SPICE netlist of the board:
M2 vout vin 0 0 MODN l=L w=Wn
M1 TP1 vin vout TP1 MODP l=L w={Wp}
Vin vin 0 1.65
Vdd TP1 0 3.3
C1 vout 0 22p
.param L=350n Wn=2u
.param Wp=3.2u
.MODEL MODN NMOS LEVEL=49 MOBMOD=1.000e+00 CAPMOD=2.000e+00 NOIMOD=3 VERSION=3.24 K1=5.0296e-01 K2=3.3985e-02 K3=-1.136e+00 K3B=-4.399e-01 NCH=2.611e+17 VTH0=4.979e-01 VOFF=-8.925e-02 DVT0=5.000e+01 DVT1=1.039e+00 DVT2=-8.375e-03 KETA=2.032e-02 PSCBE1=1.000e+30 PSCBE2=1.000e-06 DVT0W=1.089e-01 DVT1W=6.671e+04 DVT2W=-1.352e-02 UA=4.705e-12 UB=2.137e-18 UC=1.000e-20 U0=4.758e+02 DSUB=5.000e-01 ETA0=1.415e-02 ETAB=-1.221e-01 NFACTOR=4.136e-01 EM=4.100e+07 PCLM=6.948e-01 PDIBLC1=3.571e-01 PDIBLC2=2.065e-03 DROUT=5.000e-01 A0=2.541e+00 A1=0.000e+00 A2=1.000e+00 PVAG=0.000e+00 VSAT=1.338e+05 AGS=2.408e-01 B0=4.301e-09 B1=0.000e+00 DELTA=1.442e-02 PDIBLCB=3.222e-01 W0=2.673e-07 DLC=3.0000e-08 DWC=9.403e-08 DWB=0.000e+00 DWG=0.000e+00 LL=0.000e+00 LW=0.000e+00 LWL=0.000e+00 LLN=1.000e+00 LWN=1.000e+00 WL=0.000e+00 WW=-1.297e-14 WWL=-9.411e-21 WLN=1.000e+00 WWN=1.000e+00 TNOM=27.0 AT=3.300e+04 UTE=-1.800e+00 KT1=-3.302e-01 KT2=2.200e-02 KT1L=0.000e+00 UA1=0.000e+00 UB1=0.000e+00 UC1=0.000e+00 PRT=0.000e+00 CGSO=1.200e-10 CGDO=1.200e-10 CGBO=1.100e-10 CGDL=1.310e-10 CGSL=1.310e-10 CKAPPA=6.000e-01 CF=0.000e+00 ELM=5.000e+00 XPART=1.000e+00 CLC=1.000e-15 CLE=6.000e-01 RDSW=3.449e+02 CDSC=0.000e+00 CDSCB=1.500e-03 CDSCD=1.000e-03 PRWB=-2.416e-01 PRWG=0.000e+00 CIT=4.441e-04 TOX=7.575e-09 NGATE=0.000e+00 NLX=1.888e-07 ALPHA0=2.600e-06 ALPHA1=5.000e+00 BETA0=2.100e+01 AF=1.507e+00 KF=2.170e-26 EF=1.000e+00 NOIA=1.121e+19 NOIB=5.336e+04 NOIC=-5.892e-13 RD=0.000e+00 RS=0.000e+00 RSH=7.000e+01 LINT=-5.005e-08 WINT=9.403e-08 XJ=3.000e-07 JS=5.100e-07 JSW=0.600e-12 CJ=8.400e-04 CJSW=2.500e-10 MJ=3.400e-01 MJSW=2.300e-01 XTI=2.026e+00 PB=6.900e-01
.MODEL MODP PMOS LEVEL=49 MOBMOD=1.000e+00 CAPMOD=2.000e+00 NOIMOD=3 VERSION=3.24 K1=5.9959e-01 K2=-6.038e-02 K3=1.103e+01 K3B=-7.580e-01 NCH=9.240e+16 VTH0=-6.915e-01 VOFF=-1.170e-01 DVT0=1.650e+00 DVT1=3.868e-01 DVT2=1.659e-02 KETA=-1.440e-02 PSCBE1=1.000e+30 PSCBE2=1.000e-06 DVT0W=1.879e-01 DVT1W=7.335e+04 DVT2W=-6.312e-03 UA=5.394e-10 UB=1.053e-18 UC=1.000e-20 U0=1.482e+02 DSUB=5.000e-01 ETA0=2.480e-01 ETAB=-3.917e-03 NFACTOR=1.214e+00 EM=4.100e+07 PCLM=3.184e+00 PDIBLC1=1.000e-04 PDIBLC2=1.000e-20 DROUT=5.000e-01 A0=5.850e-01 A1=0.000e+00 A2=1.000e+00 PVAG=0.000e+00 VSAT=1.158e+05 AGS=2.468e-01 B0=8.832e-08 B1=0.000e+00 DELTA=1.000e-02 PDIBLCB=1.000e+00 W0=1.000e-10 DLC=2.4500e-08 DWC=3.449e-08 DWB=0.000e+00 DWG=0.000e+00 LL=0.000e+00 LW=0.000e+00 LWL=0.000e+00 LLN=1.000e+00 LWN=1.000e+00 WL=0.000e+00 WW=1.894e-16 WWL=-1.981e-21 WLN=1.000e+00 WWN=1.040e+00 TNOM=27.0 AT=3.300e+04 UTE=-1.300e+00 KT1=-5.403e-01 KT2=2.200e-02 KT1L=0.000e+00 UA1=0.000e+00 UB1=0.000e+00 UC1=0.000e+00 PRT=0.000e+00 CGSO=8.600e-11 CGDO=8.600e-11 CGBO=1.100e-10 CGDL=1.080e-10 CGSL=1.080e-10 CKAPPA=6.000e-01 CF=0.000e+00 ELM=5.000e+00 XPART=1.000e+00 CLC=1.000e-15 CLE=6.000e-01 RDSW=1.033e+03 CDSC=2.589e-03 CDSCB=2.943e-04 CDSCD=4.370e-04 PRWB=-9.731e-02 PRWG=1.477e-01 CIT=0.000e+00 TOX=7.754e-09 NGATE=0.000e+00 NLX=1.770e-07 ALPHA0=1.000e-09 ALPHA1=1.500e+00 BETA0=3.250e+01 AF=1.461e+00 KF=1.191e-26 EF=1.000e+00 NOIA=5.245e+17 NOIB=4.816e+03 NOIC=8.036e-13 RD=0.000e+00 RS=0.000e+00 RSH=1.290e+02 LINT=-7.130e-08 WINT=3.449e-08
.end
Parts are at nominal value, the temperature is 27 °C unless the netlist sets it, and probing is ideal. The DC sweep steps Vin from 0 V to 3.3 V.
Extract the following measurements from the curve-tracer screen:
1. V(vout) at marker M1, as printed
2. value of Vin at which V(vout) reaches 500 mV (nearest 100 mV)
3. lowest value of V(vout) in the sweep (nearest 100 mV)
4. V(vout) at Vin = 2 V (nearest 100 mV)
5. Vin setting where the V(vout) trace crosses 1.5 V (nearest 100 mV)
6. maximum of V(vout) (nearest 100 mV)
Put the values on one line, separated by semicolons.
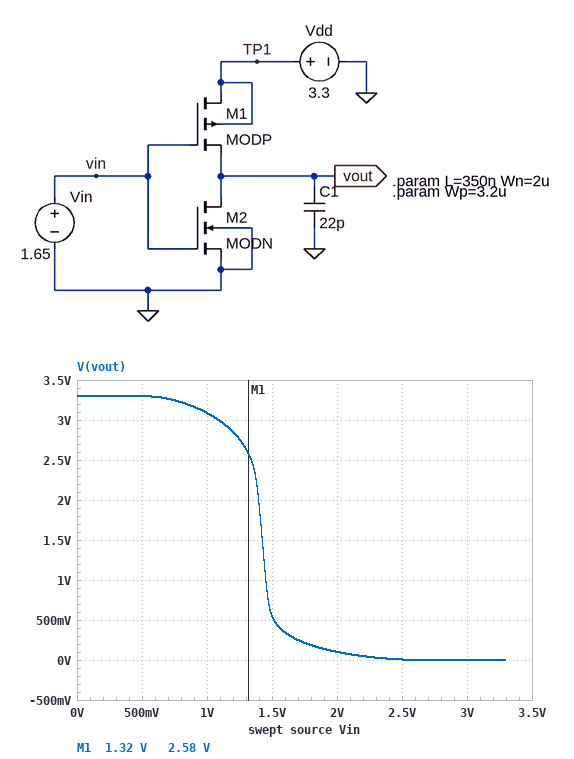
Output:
2.58 V; 1.5 V; 0 V; 100 mV; 1.4 V; 3.3 V
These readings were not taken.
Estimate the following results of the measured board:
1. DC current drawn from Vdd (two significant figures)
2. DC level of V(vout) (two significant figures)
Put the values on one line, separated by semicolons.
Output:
150 µA; 290 mV
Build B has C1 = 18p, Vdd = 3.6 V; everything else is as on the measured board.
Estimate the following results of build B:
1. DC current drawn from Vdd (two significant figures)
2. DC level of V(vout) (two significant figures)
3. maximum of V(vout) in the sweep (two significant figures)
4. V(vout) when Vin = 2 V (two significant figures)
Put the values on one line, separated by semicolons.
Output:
230 µA; 590 mV; 3.6 V; 210 mV
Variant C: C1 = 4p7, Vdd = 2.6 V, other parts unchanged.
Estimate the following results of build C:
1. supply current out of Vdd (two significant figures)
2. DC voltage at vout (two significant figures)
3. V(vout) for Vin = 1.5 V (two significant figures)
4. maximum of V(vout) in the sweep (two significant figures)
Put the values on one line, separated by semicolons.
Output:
17 µA; 27 mV; 65 mV; 2.6 V
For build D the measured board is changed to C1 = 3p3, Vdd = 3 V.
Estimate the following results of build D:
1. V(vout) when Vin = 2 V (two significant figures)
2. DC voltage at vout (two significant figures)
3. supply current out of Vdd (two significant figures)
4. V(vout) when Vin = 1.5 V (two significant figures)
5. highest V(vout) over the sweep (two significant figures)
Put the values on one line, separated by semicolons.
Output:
32 mV; 140 mV; 81 µA; 240 mV; 3.0 V
